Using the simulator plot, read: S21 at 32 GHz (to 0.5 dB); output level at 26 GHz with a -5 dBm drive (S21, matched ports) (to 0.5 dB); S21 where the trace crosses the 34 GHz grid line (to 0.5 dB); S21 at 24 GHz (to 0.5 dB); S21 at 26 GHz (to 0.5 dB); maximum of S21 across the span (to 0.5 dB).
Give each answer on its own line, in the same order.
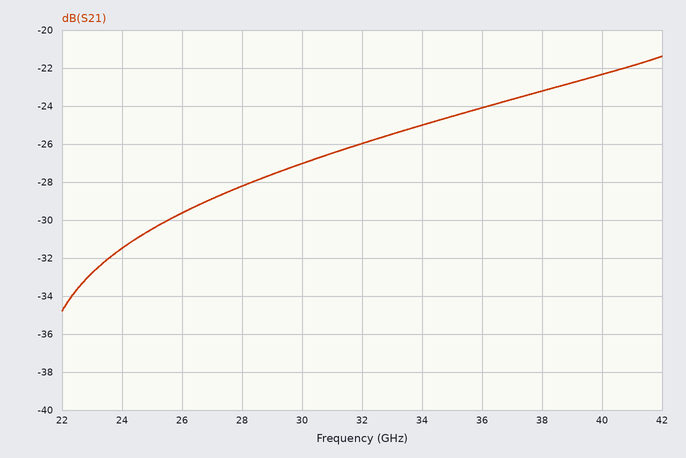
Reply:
-26.0 dB
-34.5 dBm
-25.0 dB
-31.5 dB
-29.5 dB
-21.5 dB
